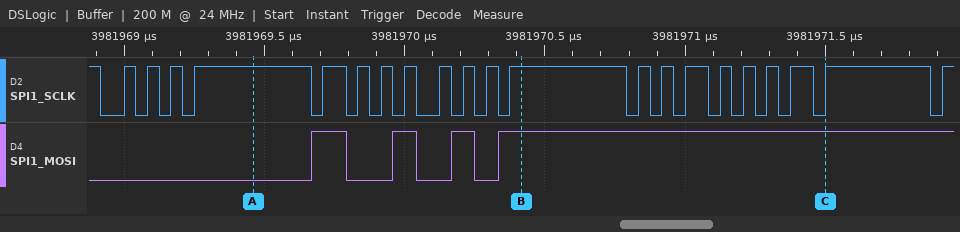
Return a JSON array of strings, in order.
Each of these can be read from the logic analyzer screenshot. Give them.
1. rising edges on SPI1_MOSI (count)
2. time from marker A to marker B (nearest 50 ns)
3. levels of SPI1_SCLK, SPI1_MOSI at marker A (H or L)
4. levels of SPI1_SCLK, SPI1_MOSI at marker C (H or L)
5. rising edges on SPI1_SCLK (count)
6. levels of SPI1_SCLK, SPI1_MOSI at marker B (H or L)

["4", "950 ns", "SPI1_SCLK=H, SPI1_MOSI=L", "SPI1_SCLK=H, SPI1_MOSI=H", "21", "SPI1_SCLK=H, SPI1_MOSI=H"]
